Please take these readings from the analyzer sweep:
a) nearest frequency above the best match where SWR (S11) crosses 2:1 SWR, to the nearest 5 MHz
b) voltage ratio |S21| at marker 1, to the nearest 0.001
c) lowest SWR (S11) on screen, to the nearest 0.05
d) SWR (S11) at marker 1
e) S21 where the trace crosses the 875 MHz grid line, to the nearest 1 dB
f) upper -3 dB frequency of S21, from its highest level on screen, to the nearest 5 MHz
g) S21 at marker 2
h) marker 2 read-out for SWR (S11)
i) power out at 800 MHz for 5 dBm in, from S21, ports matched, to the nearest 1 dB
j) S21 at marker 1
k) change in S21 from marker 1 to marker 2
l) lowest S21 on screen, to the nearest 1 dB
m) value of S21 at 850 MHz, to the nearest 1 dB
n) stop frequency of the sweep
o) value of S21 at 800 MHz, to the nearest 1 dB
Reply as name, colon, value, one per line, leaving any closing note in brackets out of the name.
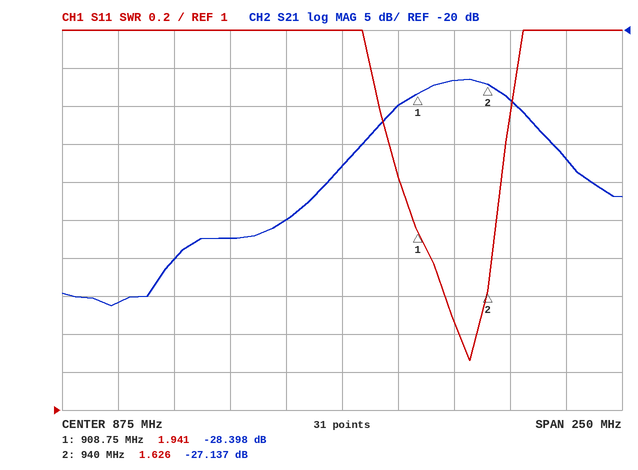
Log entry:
nearest frequency above the best match where SWR (S11) crosses 2:1 SWR, to the nearest 5 MHz: 945 MHz
voltage ratio |S21| at marker 1, to the nearest 0.001: 0.038
lowest SWR (S11) on screen, to the nearest 0.05: 1.25
SWR (S11) at marker 1: 1.941
S21 where the trace crosses the 875 MHz grid line, to the nearest 1 dB: -38 dB
upper -3 dB frequency of S21, from its highest level on screen, to the nearest 5 MHz: 950 MHz
S21 at marker 2: -27.137 dB
marker 2 read-out for SWR: 1.626
power out at 800 MHz for 5 dBm in, from S21, ports matched, to the nearest 1 dB: -45 dBm
S21 at marker 1: -28.398 dB
change in S21 from marker 1 to marker 2: 1.261 dB
lowest S21 on screen, to the nearest 1 dB: -56 dB
value of S21 at 850 MHz, to the nearest 1 dB: -45 dB
stop frequency of the sweep: 1 GHz
value of S21 at 800 MHz, to the nearest 1 dB: -50 dB
